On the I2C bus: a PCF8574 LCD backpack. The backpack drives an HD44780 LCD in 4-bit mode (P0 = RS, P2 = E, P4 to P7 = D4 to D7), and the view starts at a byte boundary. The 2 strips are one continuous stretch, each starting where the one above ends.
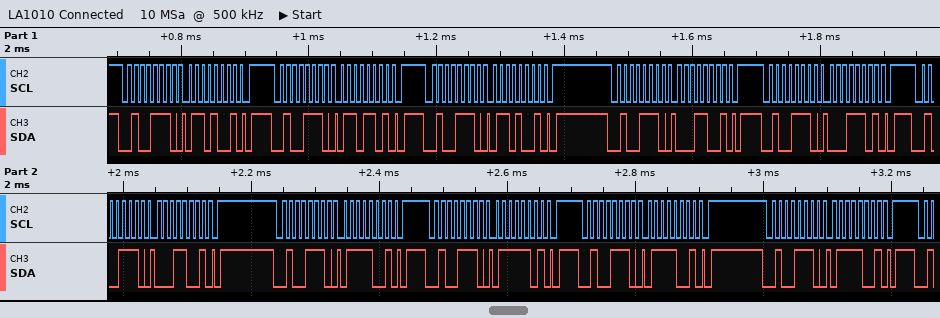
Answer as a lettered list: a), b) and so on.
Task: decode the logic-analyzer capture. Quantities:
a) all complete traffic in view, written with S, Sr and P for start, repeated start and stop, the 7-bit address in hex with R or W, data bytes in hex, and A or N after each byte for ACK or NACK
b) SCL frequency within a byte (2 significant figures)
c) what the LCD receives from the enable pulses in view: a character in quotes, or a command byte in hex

a) S 27W A 69 A P S 27W A 6D A P S 27W A 69 A P S 27W A 19 A P S 27W A 1D A P S 27W A 19 A P S 27W A 79 A P S 27W A 7D A P S 27W A 79 A P S 27W A 79 A P
b) 100 kHz
c) 'a'
